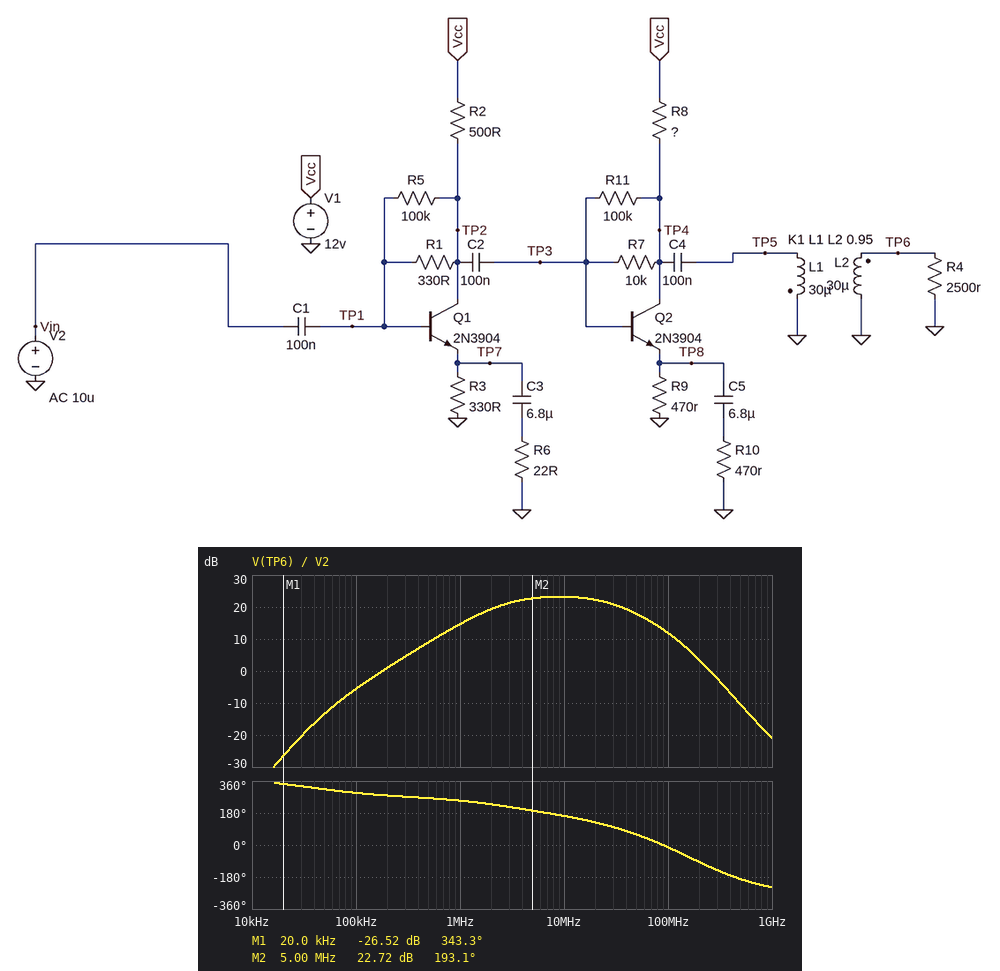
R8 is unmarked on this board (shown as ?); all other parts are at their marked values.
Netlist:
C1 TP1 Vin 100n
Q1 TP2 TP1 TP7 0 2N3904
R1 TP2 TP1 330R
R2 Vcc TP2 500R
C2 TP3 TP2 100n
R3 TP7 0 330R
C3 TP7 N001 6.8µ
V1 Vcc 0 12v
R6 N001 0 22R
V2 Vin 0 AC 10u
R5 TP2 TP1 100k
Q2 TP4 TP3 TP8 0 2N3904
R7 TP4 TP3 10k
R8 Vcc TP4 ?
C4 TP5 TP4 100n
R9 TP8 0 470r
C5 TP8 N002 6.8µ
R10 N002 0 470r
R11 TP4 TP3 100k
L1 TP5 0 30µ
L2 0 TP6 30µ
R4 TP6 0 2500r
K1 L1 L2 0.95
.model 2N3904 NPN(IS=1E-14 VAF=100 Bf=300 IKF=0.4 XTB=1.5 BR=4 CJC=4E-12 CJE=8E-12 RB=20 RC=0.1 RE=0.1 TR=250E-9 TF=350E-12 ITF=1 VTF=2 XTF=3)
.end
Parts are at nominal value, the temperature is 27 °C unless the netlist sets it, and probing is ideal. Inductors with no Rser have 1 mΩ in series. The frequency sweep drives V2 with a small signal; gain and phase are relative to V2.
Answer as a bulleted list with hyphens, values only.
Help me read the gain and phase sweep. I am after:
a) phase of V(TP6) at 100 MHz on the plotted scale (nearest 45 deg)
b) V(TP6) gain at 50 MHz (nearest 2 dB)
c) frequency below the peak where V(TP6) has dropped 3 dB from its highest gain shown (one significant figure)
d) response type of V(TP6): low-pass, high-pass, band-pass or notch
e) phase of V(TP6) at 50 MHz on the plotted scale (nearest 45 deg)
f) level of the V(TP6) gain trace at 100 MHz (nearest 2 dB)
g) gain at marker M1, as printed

- 0 deg
- 18 dB
- 2 MHz
- band-pass
- 45 deg
- 12 dB
- -26.52 dB
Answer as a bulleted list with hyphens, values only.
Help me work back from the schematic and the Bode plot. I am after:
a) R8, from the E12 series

- 680 Ω
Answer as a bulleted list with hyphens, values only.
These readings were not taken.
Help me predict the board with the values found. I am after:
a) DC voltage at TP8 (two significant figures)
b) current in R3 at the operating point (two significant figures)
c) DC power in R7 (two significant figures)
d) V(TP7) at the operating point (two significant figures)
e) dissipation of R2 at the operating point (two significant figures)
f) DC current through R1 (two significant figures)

- 4.5 V
- 14 mA
- 8.7 µW
- 4.5 V
- 92 mW
- 46 µA
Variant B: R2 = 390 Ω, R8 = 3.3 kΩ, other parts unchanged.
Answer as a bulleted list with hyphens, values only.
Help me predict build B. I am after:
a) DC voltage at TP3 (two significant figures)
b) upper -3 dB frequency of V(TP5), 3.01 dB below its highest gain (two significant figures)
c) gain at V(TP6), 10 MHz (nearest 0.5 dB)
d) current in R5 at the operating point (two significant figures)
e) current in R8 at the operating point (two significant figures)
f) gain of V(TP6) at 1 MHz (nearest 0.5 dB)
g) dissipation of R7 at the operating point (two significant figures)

- 2.1 V
- 24 MHz
- 29.5 dB
- 180 nA
- 3.0 mA
- 14.0 dB
- 820 nW
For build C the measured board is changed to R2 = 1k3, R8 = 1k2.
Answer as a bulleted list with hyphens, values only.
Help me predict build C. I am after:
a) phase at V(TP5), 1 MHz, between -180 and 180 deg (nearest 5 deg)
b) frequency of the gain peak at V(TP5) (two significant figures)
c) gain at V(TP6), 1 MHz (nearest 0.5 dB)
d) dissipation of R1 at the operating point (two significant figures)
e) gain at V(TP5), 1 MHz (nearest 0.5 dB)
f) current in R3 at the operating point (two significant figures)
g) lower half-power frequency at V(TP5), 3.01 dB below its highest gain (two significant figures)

- 75 deg
- 8.9 MHz
- 16.5 dB
- 180 nW
- 17.0 dB
- 6.9 mA
- 3.1 MHz
